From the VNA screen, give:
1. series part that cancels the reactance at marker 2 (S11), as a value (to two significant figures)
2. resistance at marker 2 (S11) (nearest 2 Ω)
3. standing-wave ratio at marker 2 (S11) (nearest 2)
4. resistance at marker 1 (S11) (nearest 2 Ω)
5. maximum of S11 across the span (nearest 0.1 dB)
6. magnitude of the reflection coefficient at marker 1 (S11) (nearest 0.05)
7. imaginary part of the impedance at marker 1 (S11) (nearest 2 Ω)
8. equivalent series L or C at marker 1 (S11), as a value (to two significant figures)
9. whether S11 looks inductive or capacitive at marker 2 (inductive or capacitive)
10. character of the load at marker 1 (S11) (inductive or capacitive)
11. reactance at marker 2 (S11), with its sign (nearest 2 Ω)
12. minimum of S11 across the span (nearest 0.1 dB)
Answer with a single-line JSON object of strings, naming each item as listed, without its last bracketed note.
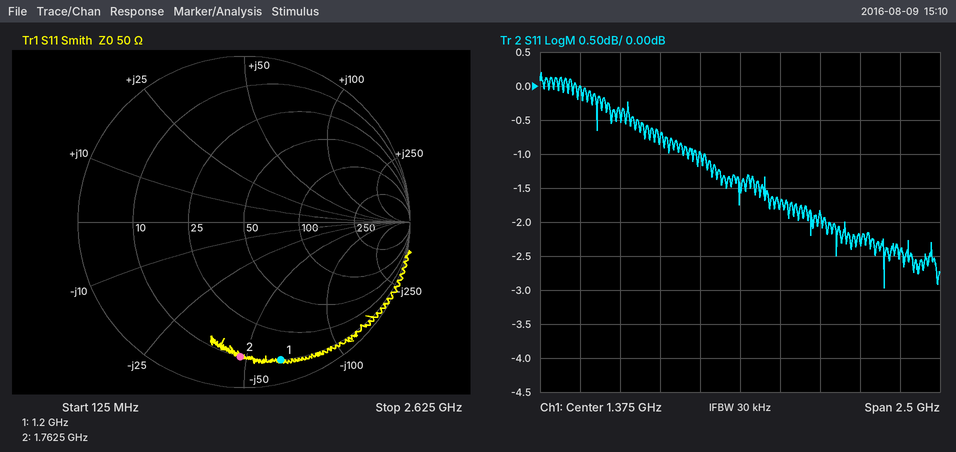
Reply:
{"series part that cancels the reactance at marker 2 (S11), as a value": "4.3 nH", "resistance at marker 2 (S11)": "10 Ω", "standing-wave ratio at marker 2 (S11)": "10", "resistance at marker 1 (S11)": "10 Ω", "maximum of S11 across the span": "0.2 dB", "magnitude of the reflection coefficient at marker 1 (S11)": "0.85", "imaginary part of the impedance at marker 1 (S11)": "-64 Ω", "equivalent series L or C at marker 1 (S11), as a value": "2.1 pF", "whether S11 looks inductive or capacitive at marker 2": "capacitive", "character of the load at marker 1 (S11)": "capacitive", "reactance at marker 2 (S11), with its sign": "-48 Ω", "minimum of S11 across the span": "-3.0 dB"}
